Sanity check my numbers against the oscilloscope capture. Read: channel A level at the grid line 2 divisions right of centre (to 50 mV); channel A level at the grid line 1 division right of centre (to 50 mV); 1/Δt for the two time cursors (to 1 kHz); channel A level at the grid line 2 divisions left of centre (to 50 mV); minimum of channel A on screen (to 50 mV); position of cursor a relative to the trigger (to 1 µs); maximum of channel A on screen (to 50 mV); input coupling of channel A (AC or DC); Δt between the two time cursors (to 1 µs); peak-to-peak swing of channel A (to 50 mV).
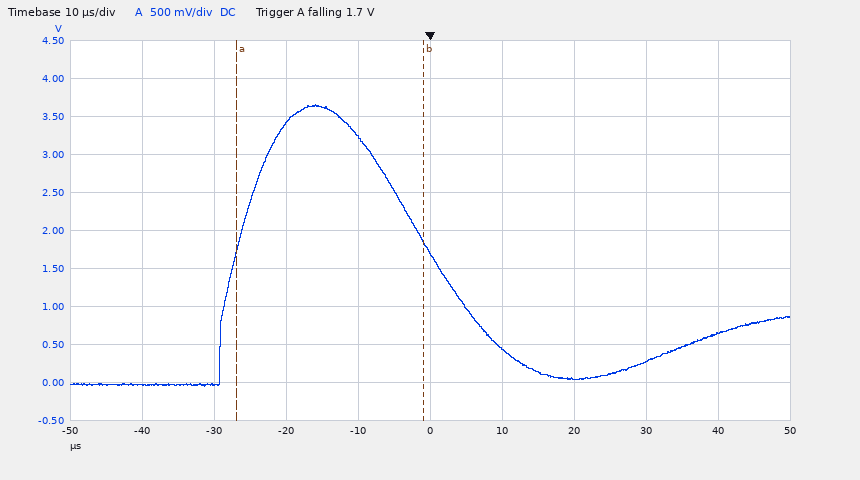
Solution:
50 mV
450 mV
38 kHz
3.40 V
-50 mV
-27 µs
3.65 V
DC
26 µs
3.70 V
